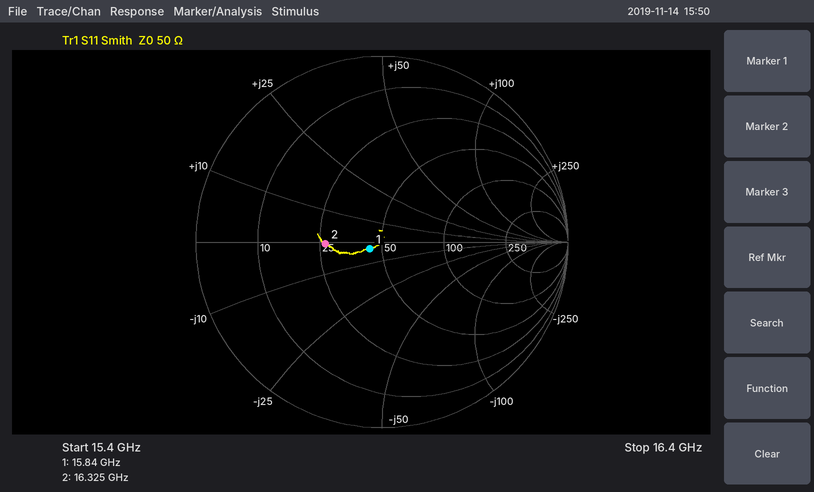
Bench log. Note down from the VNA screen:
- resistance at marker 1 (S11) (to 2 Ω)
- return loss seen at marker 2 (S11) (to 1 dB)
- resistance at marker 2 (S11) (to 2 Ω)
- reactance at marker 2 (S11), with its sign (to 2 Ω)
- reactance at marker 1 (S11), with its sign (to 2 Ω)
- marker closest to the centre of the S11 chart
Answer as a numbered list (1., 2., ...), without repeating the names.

1. 44 Ω
2. 10 dB
3. 26 Ω
4. 0 Ω
5. -4 Ω
6. marker 1
